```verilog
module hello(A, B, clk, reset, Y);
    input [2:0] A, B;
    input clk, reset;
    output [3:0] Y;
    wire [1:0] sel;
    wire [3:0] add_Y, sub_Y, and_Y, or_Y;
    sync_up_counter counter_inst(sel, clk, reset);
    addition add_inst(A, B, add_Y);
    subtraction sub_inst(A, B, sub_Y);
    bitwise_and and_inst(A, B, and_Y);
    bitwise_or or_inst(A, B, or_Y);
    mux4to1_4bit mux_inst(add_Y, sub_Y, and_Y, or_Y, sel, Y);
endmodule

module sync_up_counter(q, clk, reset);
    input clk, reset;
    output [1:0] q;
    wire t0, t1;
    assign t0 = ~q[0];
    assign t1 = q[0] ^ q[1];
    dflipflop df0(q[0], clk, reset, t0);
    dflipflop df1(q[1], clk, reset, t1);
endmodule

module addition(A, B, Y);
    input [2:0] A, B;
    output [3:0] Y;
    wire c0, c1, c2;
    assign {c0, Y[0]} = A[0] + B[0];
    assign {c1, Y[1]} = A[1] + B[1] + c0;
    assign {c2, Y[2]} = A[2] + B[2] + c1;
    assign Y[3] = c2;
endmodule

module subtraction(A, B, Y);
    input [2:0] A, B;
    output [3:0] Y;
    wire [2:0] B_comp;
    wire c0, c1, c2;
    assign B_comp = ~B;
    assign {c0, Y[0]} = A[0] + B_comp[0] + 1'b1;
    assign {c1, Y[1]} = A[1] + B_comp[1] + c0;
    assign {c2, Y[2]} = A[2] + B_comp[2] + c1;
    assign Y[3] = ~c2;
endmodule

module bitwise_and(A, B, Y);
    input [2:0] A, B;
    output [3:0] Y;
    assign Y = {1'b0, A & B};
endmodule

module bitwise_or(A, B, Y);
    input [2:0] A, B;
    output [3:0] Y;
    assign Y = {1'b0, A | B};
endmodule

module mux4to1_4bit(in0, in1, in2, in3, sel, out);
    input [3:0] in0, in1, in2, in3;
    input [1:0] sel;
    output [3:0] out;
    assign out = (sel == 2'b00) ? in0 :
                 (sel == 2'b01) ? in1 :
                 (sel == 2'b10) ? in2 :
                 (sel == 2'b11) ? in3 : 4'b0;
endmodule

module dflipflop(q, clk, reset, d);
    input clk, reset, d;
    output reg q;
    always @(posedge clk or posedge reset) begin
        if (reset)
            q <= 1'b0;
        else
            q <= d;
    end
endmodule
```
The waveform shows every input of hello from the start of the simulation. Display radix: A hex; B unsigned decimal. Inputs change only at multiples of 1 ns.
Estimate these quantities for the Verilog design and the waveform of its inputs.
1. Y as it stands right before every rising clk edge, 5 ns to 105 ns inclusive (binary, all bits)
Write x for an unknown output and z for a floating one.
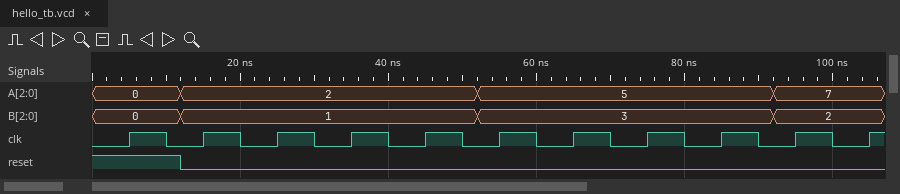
0000, 0011, 0001, 0000, 0011, 1000, 0010, 0001, 0111, 1001, 0101
